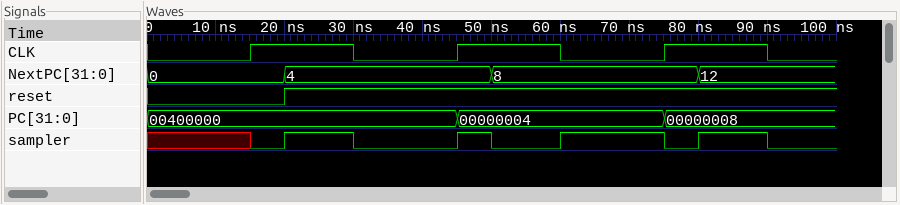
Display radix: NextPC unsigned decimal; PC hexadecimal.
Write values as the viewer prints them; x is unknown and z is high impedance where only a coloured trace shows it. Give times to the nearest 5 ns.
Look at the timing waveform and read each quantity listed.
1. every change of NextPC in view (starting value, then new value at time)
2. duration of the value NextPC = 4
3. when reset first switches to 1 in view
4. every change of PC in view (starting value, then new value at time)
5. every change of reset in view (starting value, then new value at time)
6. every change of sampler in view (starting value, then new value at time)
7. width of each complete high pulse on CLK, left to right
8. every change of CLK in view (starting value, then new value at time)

0, 4 at 20 ns, 8 at 50 ns, 12 at 80 ns
30 ns
20 ns
00400000, 00000004 at 45 ns, 00000008 at 75 ns
0, 1 at 20 ns
x, 0 at 15 ns, 1 at 20 ns, 0 at 30 ns, 1 at 45 ns, 0 at 50 ns, 1 at 60 ns, 0 at 75 ns, 1 at 80 ns, 0 at 90 ns
15 ns, 15 ns, 15 ns
0, 1 at 15 ns, 0 at 30 ns, 1 at 45 ns, 0 at 60 ns, 1 at 75 ns, 0 at 90 ns
